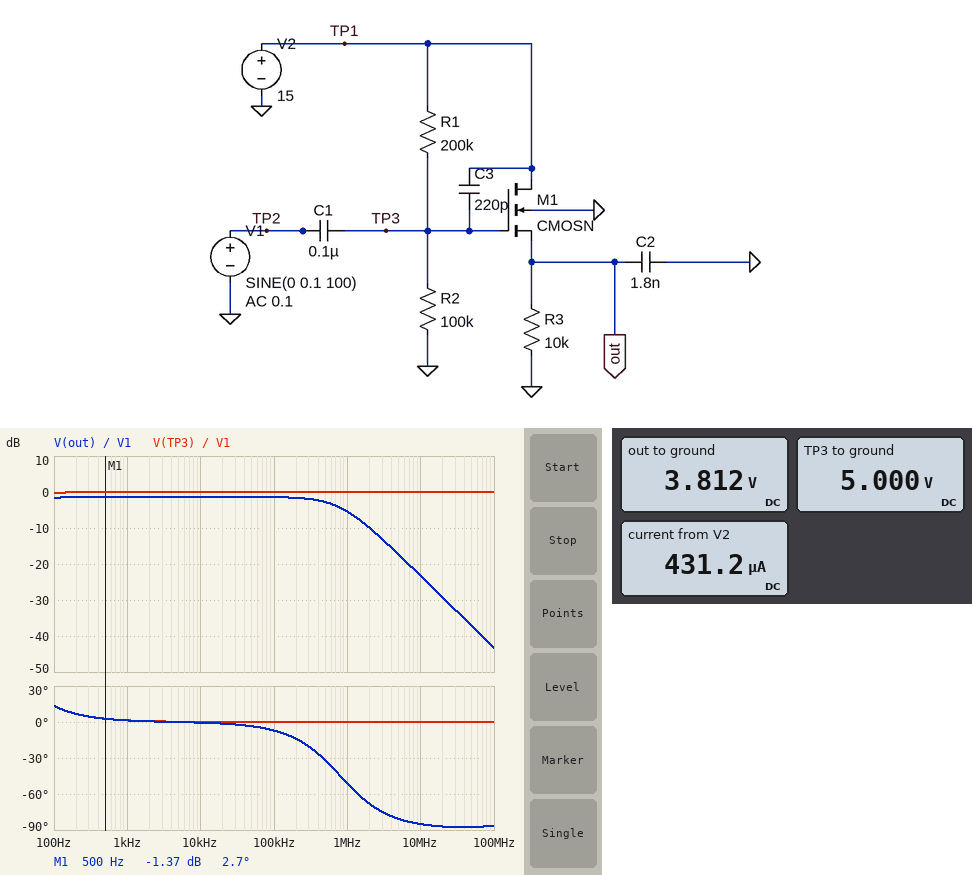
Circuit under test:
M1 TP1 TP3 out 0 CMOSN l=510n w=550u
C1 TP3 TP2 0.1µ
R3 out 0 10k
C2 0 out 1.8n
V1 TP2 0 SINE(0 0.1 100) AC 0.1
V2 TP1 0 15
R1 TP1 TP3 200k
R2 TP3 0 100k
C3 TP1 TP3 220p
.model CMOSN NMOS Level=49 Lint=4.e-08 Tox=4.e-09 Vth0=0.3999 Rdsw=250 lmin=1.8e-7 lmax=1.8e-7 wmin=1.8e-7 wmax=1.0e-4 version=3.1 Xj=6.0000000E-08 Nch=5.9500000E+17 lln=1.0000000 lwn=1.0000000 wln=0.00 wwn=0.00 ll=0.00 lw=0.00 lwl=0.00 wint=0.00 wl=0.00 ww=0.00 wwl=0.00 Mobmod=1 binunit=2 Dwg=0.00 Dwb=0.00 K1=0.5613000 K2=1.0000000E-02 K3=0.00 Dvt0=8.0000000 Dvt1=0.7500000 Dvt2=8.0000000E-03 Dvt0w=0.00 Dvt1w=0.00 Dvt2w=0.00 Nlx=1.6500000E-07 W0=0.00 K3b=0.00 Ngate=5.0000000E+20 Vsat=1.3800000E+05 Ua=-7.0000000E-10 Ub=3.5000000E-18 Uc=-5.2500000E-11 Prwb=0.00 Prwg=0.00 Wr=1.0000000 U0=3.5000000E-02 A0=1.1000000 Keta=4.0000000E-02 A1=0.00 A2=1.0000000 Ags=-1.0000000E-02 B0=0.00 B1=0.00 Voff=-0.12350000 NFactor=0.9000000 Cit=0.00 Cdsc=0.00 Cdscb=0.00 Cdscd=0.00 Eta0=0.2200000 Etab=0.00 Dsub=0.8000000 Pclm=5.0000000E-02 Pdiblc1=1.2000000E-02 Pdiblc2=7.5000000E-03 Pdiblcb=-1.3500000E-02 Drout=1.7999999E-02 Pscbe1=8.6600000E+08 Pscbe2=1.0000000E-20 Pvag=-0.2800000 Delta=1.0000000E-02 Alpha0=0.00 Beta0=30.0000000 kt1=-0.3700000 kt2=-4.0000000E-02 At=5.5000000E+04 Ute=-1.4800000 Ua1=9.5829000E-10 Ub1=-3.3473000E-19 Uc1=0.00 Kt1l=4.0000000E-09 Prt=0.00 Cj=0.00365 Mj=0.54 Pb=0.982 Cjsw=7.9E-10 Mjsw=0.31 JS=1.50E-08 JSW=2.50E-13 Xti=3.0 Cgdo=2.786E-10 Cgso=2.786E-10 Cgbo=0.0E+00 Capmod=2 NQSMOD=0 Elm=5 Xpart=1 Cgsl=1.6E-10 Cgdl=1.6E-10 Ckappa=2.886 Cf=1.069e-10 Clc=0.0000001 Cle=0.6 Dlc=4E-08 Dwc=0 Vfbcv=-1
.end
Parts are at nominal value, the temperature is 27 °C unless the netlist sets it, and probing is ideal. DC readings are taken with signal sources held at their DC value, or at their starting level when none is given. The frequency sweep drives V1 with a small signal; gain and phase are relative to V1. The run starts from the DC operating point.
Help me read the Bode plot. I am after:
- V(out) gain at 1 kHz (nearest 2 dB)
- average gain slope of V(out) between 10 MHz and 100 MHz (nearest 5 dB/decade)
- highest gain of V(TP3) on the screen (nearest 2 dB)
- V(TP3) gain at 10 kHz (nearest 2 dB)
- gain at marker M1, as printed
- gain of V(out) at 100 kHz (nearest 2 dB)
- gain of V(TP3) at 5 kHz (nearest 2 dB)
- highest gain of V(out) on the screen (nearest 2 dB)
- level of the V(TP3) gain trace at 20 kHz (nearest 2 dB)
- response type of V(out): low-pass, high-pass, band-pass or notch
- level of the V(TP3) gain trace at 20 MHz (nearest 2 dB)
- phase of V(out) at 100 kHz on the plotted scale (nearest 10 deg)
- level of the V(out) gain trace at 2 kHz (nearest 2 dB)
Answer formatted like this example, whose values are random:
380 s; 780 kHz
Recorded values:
-2 dB; -20 dB/decade; 0 dB; 0 dB; -1.37 dB; -2 dB; 0 dB; -2 dB; 0 dB; low-pass; 0 dB; -10 deg; -2 dB
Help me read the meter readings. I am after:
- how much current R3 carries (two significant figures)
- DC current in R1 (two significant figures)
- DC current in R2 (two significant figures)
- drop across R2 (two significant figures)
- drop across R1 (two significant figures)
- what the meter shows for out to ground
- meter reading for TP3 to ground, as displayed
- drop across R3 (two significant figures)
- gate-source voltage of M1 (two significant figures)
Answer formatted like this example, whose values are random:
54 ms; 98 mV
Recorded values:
380 µA; 50 µA; 50 µA; 5.0 V; 10 V; 3.812 V; 5.000 V; 3.8 V; 1.2 V
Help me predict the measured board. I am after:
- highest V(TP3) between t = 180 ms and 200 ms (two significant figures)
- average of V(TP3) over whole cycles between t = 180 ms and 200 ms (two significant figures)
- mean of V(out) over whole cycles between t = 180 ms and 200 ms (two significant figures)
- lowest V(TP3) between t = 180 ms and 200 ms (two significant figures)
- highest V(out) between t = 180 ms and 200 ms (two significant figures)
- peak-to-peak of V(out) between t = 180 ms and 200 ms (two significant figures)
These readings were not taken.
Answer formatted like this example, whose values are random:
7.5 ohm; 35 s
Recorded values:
5.1 V; 5.0 V; 3.8 V; 4.9 V; 3.9 V; 170 mV
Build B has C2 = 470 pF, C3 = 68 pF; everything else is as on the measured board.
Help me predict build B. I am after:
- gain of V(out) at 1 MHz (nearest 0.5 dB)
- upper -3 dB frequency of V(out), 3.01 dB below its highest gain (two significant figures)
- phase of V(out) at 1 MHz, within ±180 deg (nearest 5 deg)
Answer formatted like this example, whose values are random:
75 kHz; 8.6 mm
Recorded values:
-2.0 dB; 3.1 MHz; -20 deg
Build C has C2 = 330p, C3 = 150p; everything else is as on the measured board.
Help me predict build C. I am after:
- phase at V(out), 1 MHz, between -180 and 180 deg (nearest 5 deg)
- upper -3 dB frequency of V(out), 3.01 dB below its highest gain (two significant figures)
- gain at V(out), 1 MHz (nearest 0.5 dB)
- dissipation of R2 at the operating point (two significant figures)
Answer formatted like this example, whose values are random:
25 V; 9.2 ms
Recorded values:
-15 deg; 4.4 MHz; -1.5 dB; 250 µW
